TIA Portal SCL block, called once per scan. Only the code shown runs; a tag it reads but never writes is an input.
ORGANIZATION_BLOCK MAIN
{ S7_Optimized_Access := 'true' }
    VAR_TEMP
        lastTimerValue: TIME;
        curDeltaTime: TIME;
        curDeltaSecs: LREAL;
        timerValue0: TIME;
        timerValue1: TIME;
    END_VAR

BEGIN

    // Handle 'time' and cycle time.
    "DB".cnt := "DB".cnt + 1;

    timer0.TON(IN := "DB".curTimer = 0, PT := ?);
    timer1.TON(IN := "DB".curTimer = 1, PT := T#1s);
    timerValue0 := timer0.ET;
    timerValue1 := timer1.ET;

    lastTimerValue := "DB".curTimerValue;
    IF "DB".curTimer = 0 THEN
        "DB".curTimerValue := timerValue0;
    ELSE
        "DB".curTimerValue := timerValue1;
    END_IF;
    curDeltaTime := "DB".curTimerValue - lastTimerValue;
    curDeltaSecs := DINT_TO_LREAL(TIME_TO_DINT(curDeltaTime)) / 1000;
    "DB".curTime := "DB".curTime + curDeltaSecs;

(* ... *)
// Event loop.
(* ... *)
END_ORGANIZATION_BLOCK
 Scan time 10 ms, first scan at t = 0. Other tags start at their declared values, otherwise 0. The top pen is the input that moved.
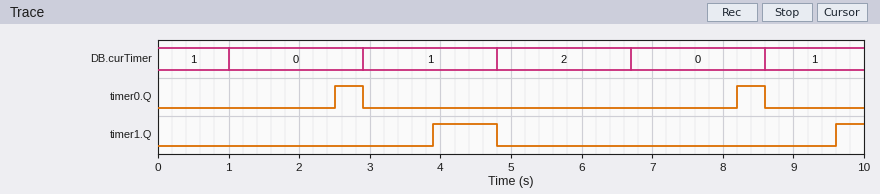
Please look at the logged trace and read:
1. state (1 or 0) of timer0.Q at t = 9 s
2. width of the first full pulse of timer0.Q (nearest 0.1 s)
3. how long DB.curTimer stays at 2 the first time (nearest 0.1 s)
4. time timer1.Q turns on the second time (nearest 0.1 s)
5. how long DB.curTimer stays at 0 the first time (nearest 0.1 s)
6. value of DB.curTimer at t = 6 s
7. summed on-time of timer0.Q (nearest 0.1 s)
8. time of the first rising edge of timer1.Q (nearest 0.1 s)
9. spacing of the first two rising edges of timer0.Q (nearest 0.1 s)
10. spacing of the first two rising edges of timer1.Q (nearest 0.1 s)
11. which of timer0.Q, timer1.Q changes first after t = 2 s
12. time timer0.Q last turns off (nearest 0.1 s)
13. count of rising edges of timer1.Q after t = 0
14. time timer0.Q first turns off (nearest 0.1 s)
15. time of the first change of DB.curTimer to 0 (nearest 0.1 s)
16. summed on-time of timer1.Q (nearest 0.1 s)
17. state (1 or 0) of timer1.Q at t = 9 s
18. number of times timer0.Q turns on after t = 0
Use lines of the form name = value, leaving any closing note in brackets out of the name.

state (1 or 0) of timer0.Q at t = 9 s = 0
width of the first full pulse of timer0.Q = 0.4 s
how long DB.curTimer stays at 2 the first time = 1.9 s
time timer1.Q turns on the second time = 9.6 s
how long DB.curTimer stays at 0 the first time = 1.9 s
value of DB.curTimer at t = 6 s = 2
summed on-time of timer0.Q = 0.8 s
time of the first rising edge of timer1.Q = 3.9 s
spacing of the first two rising edges of timer0.Q = 5.7 s
spacing of the first two rising edges of timer1.Q = 5.7 s
which of timer0.Q, timer1.Q changes first after t = 2 s = timer0.Q
time timer0.Q last turns off = 8.6 s
count of rising edges of timer1.Q after t = 0 = 2
time timer0.Q first turns off = 2.9 s
time of the first change of DB.curTimer to 0 = 1.0 s
summed on-time of timer1.Q = 1.3 s
state (1 or 0) of timer1.Q at t = 9 s = 0
number of times timer0.Q turns on after t = 0 = 2
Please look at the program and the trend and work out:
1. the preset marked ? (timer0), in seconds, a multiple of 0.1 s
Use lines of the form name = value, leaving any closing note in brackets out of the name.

the preset marked ? (timer0), in seconds, a multiple of 0.1 s = 1.5 s
